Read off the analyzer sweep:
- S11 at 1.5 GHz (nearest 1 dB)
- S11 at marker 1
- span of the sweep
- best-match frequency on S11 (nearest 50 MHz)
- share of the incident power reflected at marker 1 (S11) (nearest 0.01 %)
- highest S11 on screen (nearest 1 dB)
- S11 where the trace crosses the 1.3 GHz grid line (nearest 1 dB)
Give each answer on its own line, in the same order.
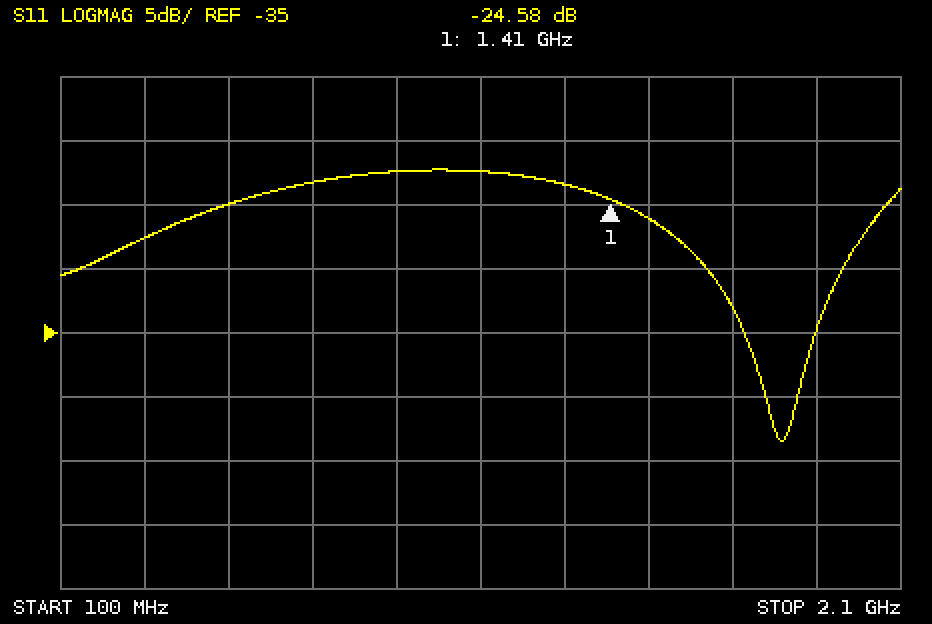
-26 dB
-24.58 dB
2 GHz
1.80 GHz
0.35 %
-22 dB
-23 dB
